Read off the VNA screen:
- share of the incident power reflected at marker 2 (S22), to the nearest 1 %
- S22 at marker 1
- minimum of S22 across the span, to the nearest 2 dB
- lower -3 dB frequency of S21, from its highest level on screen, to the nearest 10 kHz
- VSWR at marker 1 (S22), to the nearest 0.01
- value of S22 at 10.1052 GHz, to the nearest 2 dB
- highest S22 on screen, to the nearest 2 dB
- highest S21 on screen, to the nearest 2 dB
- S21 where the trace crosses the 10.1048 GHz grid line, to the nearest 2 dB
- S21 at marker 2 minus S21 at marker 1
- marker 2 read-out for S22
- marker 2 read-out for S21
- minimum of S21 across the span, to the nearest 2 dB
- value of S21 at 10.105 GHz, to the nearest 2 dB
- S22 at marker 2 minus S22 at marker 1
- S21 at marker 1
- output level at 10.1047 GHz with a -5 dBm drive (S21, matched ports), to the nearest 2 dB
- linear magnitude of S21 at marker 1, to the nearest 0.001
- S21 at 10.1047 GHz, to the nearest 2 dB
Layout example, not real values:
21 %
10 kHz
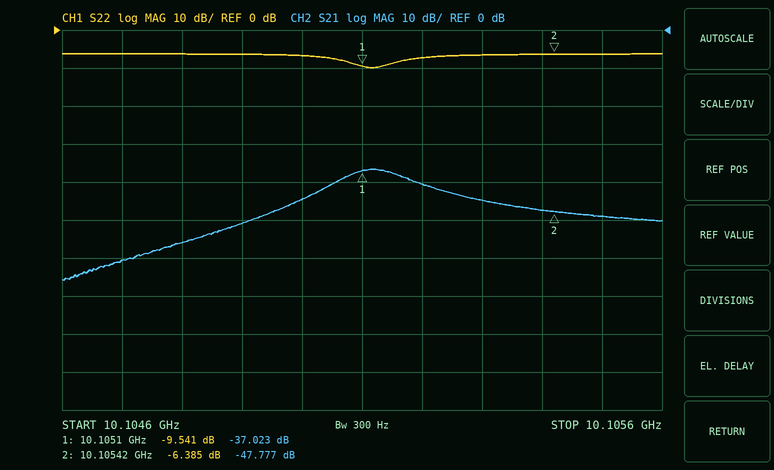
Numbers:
23 %
-9.541 dB
-10 dB
10.10506 GHz
2.00
-8 dB
-6 dB
-36 dB
-56 dB
-10.754 dB
-6.385 dB
-47.777 dB
-66 dB
-44 dB
3.156 dB
-37.023 dB
-66 dBm
0.014
-60 dB
